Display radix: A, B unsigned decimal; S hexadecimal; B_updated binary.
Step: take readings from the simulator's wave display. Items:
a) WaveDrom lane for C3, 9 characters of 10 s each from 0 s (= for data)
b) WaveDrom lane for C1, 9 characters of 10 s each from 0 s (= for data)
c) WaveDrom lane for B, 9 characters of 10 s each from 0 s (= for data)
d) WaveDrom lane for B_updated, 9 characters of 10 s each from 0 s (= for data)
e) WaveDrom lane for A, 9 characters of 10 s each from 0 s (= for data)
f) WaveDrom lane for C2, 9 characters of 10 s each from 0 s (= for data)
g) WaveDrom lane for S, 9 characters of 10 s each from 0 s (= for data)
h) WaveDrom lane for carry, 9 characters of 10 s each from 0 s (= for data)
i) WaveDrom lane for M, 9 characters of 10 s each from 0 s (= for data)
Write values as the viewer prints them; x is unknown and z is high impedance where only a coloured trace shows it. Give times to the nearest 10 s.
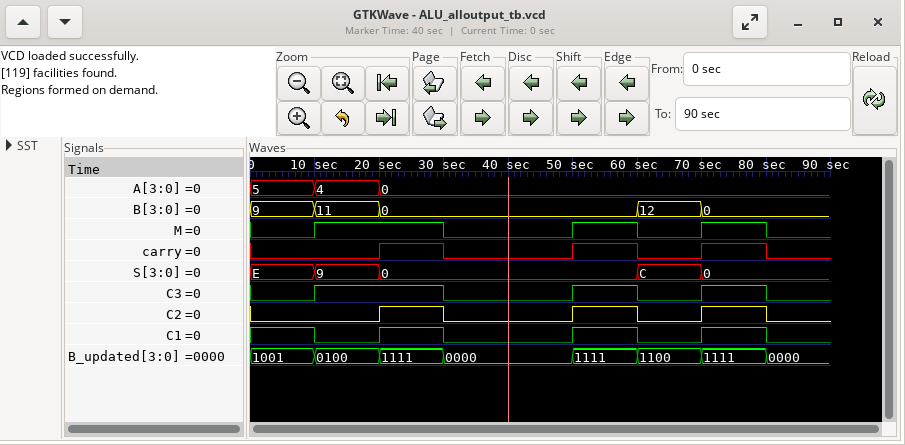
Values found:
{name: 'C3', wave: '01.0.1010'}
{name: 'C1', wave: '1010.1010'}
{name: 'B', wave: '===...==.', data: '9 11 0 12 0'}
{name: 'B_updated', wave: '====.====', data: '1001 0100 1111 0000 1111 1100 1111 0000'}
{name: 'A', wave: '===......', data: '5 4 0'}
{name: 'C2', wave: '0.10.1010'}
{name: 'S', wave: '===...==.', data: 'E 9 0 C 0'}
{name: 'carry', wave: '0.10.1010'}
{name: 'M', wave: '01.0.1010'}
